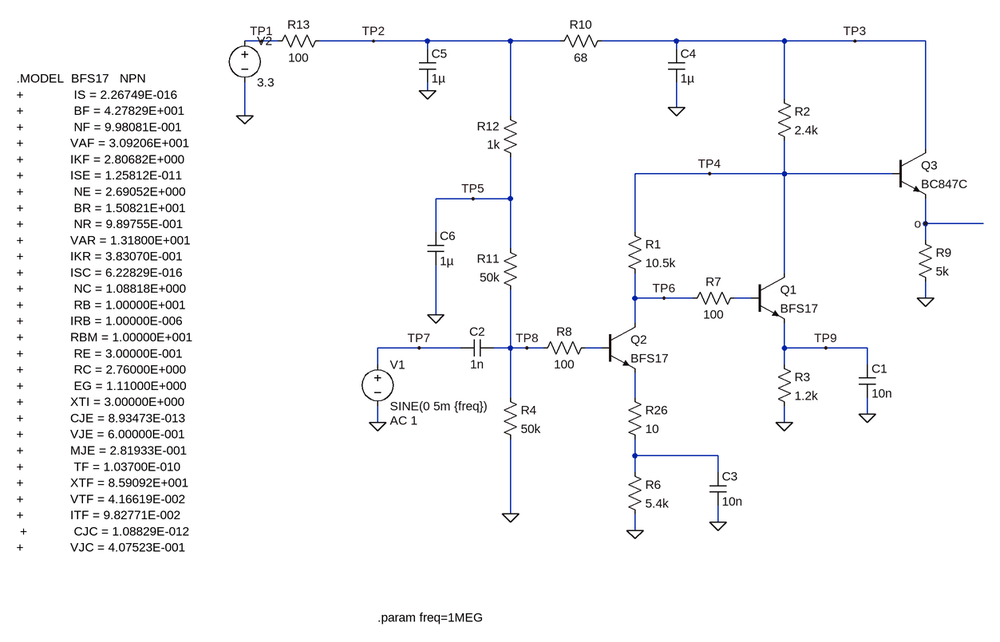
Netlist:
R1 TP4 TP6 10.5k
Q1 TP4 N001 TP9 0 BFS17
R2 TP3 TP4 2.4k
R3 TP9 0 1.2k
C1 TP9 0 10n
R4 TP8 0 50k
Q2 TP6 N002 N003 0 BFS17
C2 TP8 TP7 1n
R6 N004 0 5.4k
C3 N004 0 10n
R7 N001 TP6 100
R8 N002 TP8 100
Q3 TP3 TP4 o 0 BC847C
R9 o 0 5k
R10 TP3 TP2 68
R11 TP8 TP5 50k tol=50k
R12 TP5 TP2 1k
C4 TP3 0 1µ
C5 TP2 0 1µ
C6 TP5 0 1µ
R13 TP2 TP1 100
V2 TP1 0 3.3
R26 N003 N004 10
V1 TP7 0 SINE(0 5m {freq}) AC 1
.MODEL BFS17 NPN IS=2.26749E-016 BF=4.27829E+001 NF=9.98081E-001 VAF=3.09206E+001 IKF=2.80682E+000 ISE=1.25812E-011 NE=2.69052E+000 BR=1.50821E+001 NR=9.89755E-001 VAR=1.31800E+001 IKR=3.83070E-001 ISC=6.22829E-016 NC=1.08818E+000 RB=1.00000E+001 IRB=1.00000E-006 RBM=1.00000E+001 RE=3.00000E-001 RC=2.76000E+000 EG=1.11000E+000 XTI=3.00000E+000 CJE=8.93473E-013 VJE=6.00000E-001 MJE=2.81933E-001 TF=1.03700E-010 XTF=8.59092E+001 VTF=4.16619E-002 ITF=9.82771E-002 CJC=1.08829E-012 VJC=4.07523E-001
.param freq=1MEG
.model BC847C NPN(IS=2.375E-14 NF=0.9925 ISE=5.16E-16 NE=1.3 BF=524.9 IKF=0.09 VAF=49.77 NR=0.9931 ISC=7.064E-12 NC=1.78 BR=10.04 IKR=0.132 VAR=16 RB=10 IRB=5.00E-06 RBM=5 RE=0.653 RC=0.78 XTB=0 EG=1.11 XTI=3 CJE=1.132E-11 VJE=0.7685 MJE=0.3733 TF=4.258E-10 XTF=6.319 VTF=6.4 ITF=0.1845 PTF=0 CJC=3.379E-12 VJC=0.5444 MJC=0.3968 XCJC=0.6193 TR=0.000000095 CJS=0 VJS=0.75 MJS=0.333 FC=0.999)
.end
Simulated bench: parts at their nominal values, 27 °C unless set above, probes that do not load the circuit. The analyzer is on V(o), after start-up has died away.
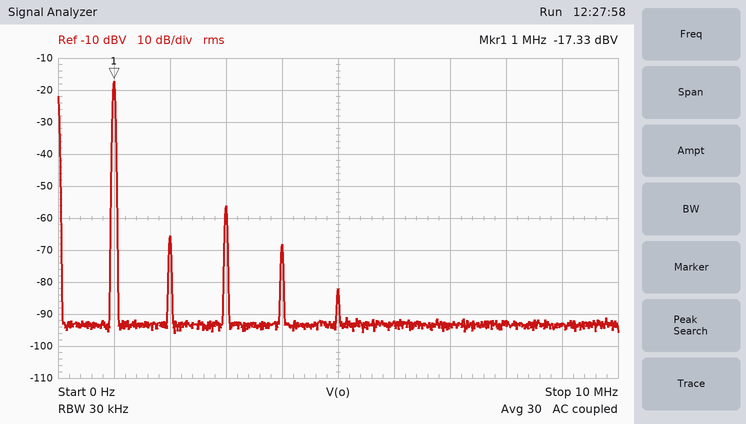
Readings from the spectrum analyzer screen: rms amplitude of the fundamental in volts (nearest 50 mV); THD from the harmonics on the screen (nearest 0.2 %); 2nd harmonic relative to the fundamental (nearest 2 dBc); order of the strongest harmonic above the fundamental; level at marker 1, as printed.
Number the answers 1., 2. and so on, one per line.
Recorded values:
1. 150 mV
2. 1.2 %
3. -48 dBc
4. 3
5. -17.33 dBV
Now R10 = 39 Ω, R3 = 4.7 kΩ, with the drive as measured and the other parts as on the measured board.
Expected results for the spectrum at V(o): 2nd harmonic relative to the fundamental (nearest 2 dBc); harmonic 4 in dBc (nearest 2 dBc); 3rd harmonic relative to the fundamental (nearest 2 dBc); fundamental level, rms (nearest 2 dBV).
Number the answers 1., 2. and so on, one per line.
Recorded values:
1. -22 dBc
2. -34 dBc
3. -26 dBc
4. -18 dBV
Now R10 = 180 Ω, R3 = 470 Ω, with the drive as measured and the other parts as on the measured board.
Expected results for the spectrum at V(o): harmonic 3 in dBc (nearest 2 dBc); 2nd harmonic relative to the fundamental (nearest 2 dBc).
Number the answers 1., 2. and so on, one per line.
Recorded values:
1. -42 dBc
2. -36 dBc
